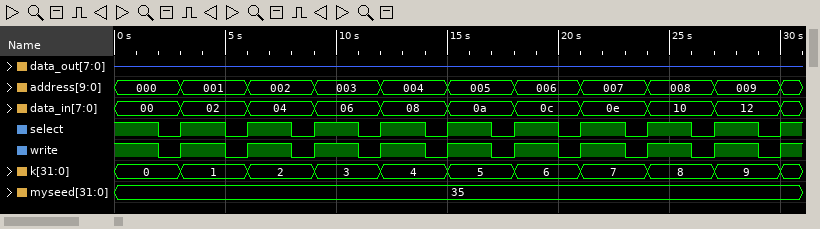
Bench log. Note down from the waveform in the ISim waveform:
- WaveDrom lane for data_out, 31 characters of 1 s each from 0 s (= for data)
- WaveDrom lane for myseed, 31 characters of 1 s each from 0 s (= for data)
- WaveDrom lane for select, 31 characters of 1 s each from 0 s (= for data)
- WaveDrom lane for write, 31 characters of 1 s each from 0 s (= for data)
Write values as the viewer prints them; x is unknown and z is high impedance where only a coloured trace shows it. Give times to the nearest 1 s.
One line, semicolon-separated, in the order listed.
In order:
{name: 'data_out', wave: 'z..............................'}; {name: 'myseed', wave: '=..............................', data: '35'}; {name: 'select', wave: '1.01.01.01.01.01.01.01.01.01.01'}; {name: 'write', wave: '1.01.01.01.01.01.01.01.01.01.01'}
